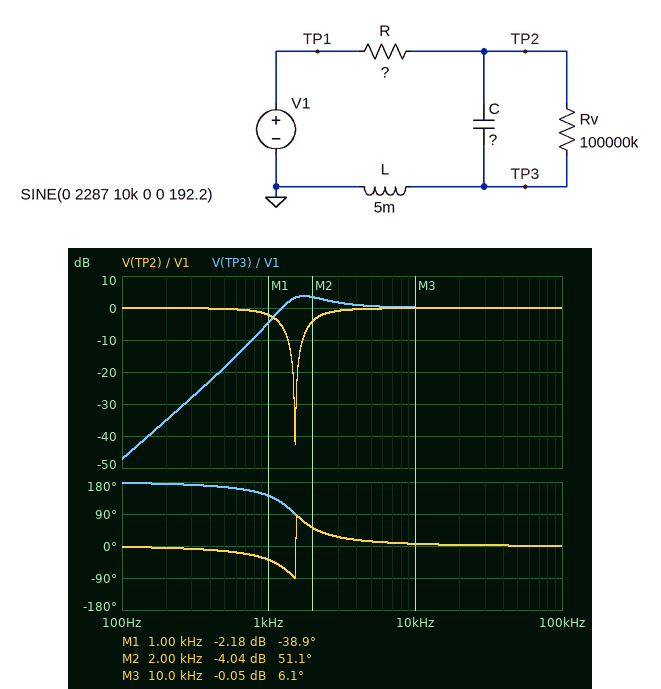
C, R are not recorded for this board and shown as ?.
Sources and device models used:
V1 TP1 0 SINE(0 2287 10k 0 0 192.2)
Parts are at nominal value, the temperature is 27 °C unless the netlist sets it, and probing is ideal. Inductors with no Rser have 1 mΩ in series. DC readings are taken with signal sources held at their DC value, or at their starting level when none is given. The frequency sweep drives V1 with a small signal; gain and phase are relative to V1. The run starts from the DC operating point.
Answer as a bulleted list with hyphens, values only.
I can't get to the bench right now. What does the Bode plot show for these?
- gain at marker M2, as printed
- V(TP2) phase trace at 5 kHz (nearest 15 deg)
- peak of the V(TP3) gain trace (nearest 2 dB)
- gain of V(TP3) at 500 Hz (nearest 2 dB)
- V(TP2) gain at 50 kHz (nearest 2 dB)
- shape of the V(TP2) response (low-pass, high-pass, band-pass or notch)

- -4.04 dB
- 15 deg
- 4 dB
- -18 dB
- 0 dB
- notch
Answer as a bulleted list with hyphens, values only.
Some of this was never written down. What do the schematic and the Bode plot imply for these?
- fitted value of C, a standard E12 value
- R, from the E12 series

- 2.2 µF
- 33 Ω
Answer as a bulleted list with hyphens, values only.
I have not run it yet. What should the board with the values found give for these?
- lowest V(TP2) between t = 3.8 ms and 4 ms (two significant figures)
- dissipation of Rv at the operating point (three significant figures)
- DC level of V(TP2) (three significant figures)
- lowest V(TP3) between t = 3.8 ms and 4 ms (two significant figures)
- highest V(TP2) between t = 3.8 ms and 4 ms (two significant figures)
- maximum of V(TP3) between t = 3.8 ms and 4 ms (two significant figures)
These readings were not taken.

- -2.3 kV
- 2.34 mW
- -483 V
- -2.3 kV
- 2.3 kV
- 2.3 kV
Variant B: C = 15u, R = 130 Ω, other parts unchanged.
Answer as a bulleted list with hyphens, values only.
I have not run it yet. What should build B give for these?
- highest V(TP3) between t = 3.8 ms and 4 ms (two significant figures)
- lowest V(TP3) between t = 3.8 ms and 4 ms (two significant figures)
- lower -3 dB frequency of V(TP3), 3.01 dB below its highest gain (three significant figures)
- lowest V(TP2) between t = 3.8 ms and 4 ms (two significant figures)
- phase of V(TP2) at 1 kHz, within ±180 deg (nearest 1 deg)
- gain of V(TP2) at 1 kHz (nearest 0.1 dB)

- 2.1 kV
- -2.1 kV
- 4.06 kHz
- -2.2 kV
- 81 deg
- -16.0 dB
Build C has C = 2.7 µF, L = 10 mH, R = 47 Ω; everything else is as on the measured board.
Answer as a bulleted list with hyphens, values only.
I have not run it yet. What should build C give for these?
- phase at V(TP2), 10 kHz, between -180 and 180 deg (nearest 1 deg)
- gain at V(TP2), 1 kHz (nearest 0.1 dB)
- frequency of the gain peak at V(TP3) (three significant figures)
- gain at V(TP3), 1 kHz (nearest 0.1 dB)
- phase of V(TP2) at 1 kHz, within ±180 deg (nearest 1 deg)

- 4 deg
- -21.7 dB
- 1.16 kHz
- 2.5 dB
- 85 deg
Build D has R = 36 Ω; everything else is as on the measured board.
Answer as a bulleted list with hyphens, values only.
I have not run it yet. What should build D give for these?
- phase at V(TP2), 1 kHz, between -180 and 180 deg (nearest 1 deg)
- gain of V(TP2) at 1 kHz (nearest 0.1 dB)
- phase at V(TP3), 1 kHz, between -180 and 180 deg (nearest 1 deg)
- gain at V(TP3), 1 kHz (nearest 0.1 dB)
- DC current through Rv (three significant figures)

- -41 deg
- -2.5 dB
- 139 deg
- -4.8 dB
- 4.83 µA
